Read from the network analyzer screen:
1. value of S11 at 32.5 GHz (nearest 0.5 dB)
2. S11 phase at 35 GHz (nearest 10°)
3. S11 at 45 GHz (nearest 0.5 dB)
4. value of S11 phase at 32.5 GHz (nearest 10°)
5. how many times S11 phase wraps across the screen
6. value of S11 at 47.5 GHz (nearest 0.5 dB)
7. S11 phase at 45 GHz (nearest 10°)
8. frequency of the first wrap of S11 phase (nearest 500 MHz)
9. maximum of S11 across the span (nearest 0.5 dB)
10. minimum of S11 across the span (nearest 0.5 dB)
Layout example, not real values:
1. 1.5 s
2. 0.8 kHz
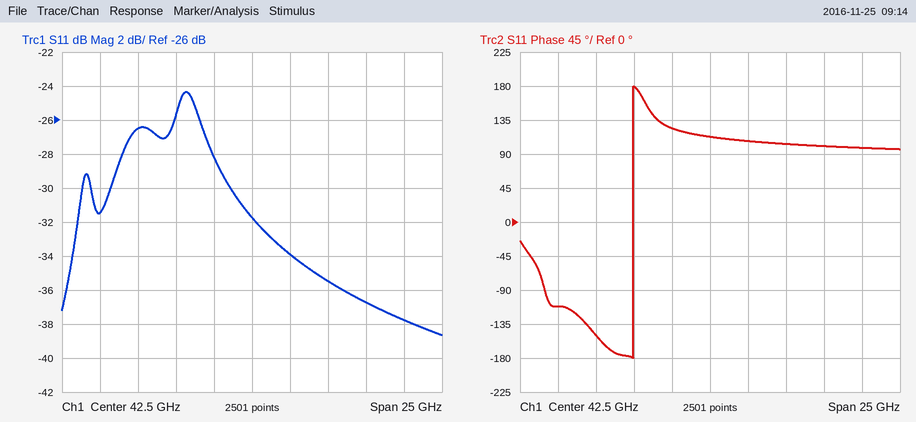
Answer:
1. -31.5 dB
2. -150°
3. -34.0 dB
4. -110°
5. 1
6. -35.5 dB
7. 110°
8. 37.5 GHz
9. -24.5 dB
10. -38.5 dB
